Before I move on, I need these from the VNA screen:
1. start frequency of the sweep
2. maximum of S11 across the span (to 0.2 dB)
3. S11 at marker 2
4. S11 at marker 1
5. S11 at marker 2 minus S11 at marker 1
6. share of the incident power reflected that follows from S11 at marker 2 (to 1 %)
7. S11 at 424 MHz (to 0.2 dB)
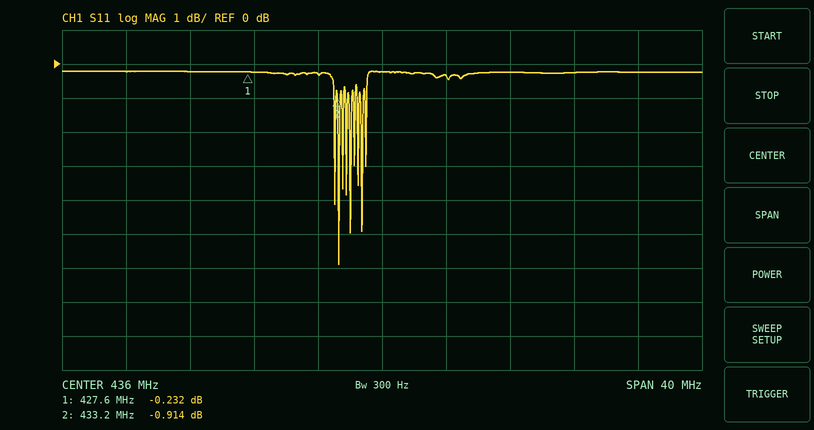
416 MHz
-0.2 dB
-0.914 dB
-0.232 dB
-0.682 dB
81 %
-0.2 dB
